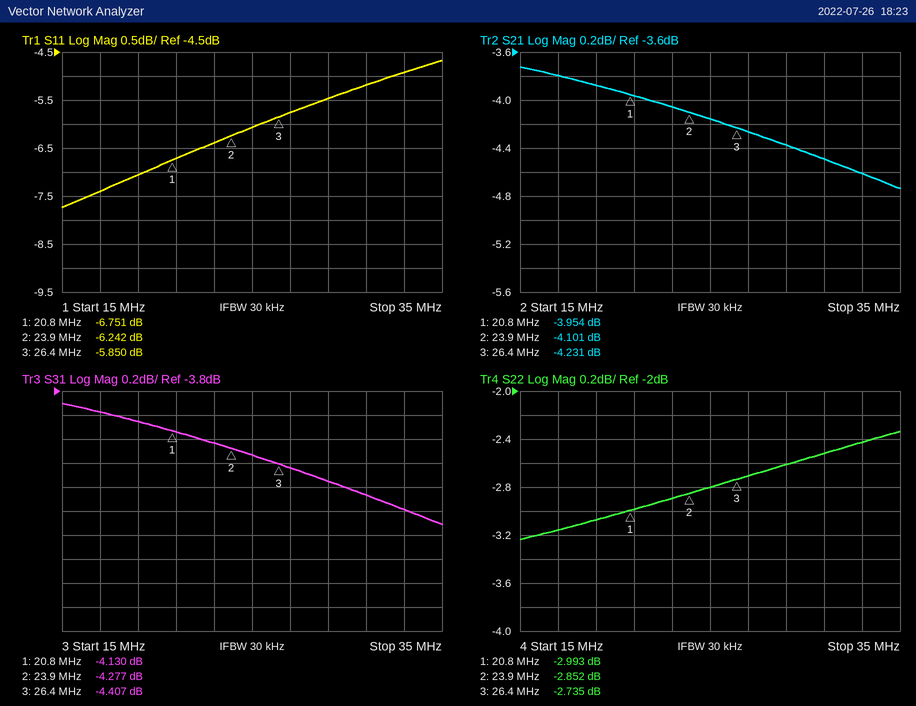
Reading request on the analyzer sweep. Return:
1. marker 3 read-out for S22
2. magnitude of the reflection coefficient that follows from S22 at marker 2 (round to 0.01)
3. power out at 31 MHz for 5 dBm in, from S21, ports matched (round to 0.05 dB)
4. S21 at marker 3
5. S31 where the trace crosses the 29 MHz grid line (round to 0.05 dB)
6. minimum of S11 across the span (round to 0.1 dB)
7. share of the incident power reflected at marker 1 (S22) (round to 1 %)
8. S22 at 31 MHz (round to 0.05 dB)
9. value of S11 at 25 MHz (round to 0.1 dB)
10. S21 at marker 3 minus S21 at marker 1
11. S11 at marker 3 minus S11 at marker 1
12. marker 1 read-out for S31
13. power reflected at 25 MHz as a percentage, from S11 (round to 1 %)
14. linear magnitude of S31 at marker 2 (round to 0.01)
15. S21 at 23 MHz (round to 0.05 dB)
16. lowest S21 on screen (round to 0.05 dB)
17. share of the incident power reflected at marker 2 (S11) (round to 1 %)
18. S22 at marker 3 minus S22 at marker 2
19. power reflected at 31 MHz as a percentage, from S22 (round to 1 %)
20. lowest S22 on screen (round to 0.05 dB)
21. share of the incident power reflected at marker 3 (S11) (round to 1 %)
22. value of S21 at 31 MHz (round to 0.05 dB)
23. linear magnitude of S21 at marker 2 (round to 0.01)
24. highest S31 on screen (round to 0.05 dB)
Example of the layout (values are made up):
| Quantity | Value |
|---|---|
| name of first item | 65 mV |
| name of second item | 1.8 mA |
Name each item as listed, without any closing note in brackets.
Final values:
| Quantity | Value |
|---|---|
| marker 3 read-out for S22 | -2.735 dB |
| magnitude of the reflection coefficient that follows from S22 at marker 2 | 0.72 |
| power out at 31 MHz for 5 dBm in, from S21, ports matched | 0.50 dBm |
| S21 at marker 3 | -4.231 dB |
| S31 where the trace crosses the 29 MHz grid line | -4.55 dB |
| minimum of S11 across the span | -7.7 dB |
| share of the incident power reflected at marker 1 (S22) | 50 % |
| S22 at 31 MHz | -2.50 dB |
| value of S11 at 25 MHz | -6.1 dB |
| S21 at marker 3 minus S21 at marker 1 | -0.277 dB |
| S11 at marker 3 minus S11 at marker 1 | 0.901 dB |
| marker 1 read-out for S31 | -4.130 dB |
| power reflected at 25 MHz as a percentage, from S11 | 25 % |
| linear magnitude of S31 at marker 2 | 0.61 |
| S21 at 23 MHz | -4.05 dB |
| lowest S21 on screen | -4.75 dB |
| share of the incident power reflected at marker 2 (S11) | 24 % |
| S22 at marker 3 minus S22 at marker 2 | 0.117 dB |
| power reflected at 31 MHz as a percentage, from S22 | 56 % |
| lowest S22 on screen | -3.25 dB |
| share of the incident power reflected at marker 3 (S11) | 26 % |
| value of S21 at 31 MHz | -4.50 dB |
| linear magnitude of S21 at marker 2 | 0.62 |
| highest S31 on screen | -3.90 dB |
